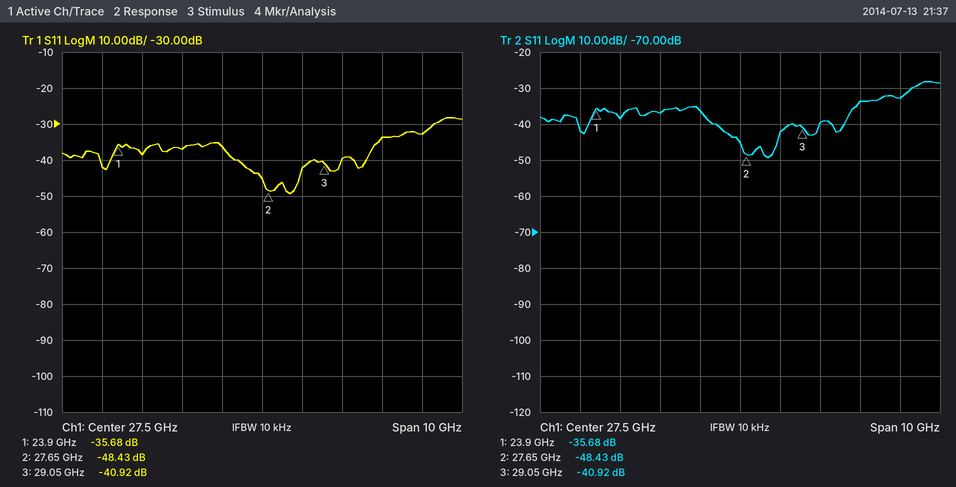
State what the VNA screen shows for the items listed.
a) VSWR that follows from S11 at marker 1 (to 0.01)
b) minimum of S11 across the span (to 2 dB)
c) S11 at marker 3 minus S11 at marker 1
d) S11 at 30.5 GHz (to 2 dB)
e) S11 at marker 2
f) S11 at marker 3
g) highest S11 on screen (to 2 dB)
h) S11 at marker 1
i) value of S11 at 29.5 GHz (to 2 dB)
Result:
1.03
-50 dB
-5.24 dB
-34 dB
-48.43 dB
-40.92 dB
-28 dB
-35.68 dB
-40 dB
